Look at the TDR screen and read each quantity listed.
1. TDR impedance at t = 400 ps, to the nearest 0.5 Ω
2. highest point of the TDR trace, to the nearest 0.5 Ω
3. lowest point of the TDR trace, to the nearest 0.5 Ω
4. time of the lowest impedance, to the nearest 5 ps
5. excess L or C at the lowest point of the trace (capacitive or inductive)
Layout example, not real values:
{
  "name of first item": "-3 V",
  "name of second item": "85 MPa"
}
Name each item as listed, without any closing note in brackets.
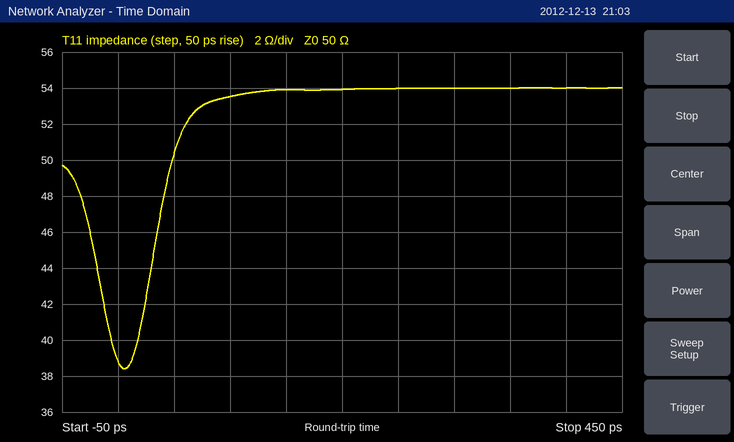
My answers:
{
  "TDR impedance at t = 400 ps, to the nearest 0.5 Ω": "54.0 Ω",
  "highest point of the TDR trace, to the nearest 0.5 Ω": "54.0 Ω",
  "lowest point of the TDR trace, to the nearest 0.5 Ω": "38.5 Ω",
  "time of the lowest impedance, to the nearest 5 ps": "5 ps",
  "excess L or C at the lowest point of the trace": "capacitive"
}
